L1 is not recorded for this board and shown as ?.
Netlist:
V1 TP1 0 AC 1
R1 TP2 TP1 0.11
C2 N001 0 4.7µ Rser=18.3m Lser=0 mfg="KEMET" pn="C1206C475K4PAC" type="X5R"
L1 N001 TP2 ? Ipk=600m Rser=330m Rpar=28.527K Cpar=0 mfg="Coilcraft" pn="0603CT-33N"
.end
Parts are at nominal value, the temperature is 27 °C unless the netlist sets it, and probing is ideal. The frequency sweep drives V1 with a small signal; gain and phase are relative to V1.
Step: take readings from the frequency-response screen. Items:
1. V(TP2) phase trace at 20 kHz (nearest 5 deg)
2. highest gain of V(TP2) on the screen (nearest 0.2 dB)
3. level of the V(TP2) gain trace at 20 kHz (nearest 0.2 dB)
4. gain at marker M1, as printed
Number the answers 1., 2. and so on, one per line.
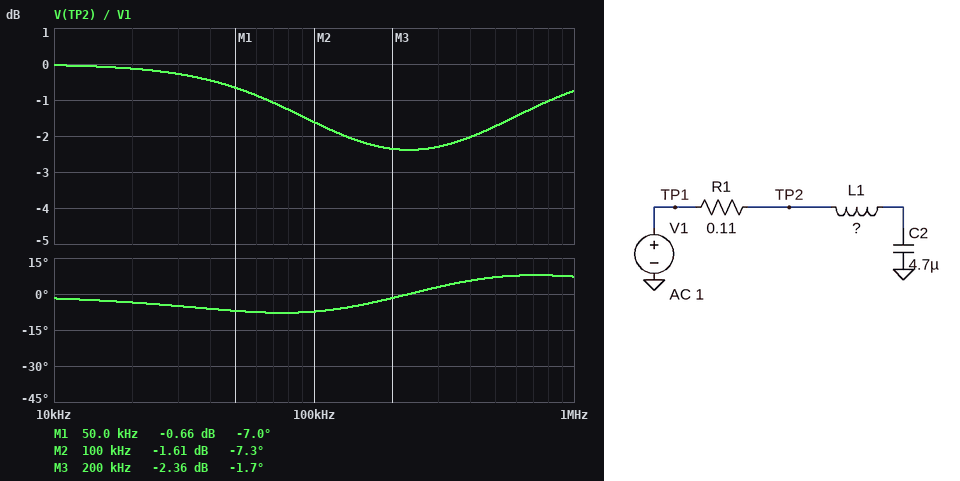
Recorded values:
1. -5 deg
2. 0 dB
3. -0.2 dB
4. -0.66 dB
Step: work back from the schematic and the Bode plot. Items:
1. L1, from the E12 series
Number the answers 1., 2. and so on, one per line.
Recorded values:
1. 100 nH
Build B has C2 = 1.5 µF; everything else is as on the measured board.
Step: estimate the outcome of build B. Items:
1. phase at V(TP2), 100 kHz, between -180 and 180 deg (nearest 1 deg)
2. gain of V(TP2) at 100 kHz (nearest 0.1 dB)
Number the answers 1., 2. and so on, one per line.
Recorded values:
1. -5 deg
2. -0.3 dB
